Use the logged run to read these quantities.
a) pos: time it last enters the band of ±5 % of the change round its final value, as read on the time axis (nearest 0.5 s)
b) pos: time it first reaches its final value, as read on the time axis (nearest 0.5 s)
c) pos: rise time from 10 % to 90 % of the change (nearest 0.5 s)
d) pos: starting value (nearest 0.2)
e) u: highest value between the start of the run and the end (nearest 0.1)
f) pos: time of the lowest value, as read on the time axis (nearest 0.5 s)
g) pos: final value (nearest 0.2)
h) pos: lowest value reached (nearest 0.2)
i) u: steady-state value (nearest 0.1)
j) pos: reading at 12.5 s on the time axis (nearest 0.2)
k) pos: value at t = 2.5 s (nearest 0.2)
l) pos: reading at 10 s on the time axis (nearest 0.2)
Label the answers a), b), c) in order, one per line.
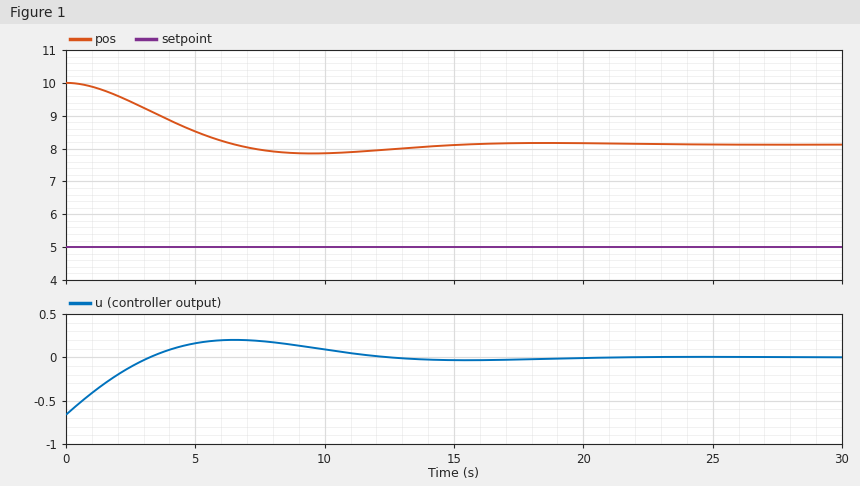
a) 13.5 s
b) 6.5 s
c) 4.5 s
d) 10.0
e) 0.2
f) 9.5 s
g) 8.2
h) 7.8
i) 0.0
j) 8.0
k) 9.4
l) 7.8
